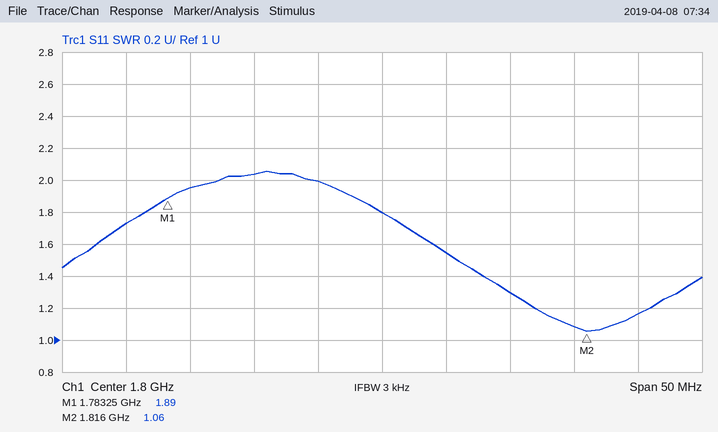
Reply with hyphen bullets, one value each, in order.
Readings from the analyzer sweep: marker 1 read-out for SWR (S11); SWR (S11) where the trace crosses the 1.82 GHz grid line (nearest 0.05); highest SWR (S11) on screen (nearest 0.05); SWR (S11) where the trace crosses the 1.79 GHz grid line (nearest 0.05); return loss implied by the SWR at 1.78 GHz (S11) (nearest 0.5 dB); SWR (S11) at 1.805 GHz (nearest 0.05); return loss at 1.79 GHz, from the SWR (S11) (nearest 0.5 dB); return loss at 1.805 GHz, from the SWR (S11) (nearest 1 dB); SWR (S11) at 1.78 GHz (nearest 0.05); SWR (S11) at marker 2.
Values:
- 1.89
- 1.15
- 2.05
- 2.05
- 11.5 dB
- 1.55
- 9.5 dB
- 13 dB
- 1.75
- 1.06
